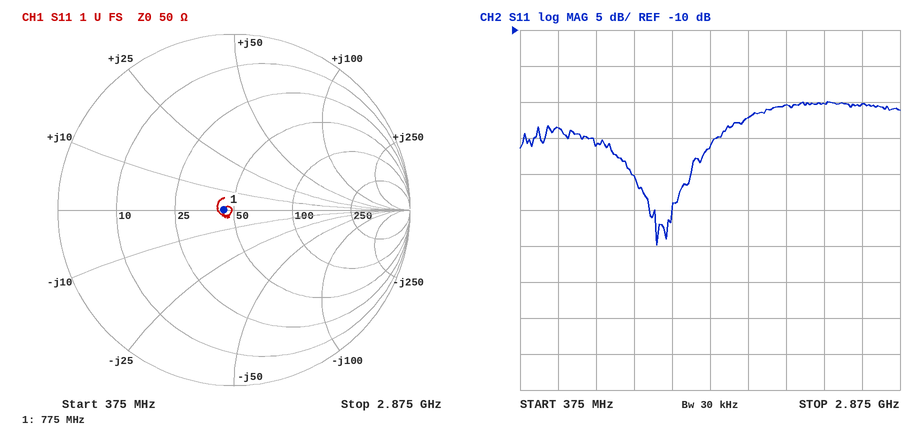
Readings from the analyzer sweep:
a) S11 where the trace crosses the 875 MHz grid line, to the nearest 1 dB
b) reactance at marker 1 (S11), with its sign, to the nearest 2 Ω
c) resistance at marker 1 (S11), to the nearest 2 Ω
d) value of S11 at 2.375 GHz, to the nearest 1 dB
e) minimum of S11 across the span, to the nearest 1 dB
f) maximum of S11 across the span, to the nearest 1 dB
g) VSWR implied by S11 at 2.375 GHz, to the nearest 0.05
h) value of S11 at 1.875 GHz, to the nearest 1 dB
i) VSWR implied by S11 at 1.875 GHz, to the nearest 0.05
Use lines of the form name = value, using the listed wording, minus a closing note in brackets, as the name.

S11 where the trace crosses the 875 MHz grid line, to the nearest 1 dB = -26 dB
reactance at marker 1 (S11), with its sign, to the nearest 2 Ω = 0 Ω
resistance at marker 1 (S11), to the nearest 2 Ω = 44 Ω
value of S11 at 2.375 GHz, to the nearest 1 dB = -20 dB
minimum of S11 across the span, to the nearest 1 dB = -40 dB
maximum of S11 across the span, to the nearest 1 dB = -20 dB
VSWR implied by S11 at 2.375 GHz, to the nearest 0.05 = 1.20
value of S11 at 1.875 GHz, to the nearest 1 dB = -22 dB
VSWR implied by S11 at 1.875 GHz, to the nearest 0.05 = 1.15
